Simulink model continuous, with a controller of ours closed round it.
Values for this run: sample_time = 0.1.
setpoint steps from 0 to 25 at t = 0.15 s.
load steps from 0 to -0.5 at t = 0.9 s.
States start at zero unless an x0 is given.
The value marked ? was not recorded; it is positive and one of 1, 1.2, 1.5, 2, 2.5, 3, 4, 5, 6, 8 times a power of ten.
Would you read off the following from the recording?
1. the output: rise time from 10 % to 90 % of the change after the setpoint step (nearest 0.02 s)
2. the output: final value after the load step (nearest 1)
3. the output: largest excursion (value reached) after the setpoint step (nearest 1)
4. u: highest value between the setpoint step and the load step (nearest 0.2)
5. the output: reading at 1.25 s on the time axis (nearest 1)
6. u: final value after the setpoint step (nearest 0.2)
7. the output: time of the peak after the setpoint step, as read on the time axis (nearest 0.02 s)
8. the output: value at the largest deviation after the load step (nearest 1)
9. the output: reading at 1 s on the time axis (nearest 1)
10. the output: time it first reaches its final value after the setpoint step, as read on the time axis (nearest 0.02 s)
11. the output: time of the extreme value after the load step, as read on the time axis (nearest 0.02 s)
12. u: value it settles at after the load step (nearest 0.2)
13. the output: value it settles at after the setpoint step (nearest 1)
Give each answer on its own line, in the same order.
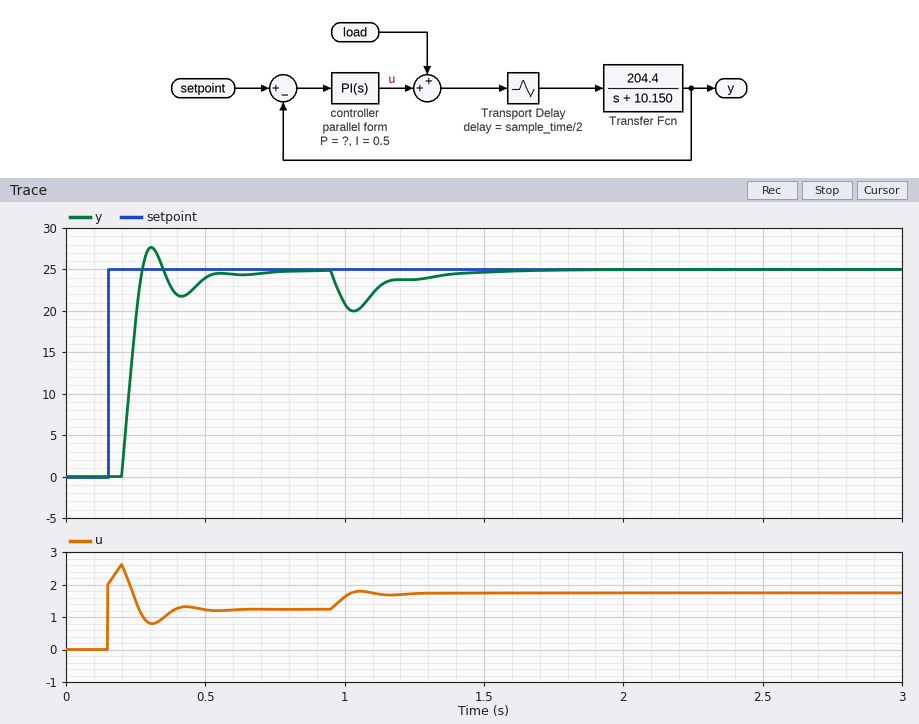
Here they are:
0.06 s
25
28
2.6
24
1.2
0.30 s
20
21
0.28 s
1.04 s
1.8
25
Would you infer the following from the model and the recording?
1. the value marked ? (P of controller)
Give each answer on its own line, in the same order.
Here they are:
0.08
